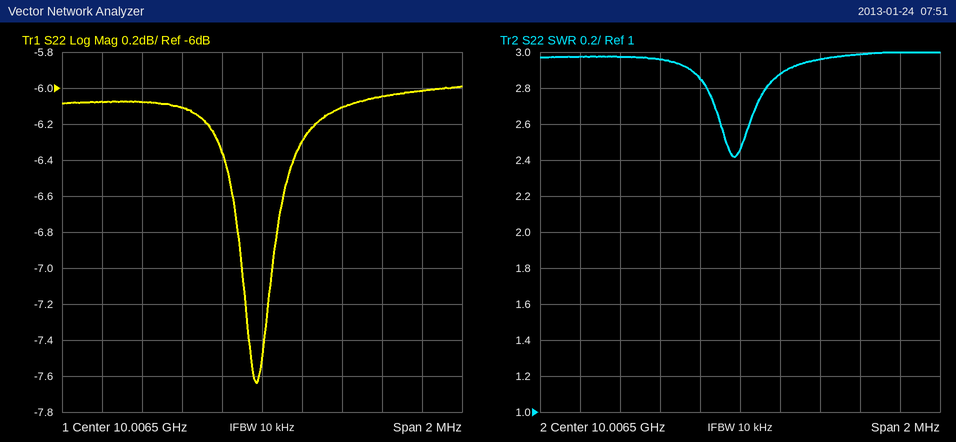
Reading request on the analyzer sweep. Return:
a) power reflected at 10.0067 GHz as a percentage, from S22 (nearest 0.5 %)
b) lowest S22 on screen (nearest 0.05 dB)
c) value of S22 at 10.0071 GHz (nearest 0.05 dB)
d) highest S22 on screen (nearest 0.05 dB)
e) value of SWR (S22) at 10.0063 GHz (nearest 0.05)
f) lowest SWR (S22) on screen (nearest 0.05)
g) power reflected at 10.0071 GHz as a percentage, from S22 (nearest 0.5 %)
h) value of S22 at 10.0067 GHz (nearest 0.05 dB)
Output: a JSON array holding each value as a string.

["23.5 %", "-7.65 dB", "-6.05 dB", "-6.00 dB", "2.85", "2.40", "25.0 %", "-6.30 dB"]
